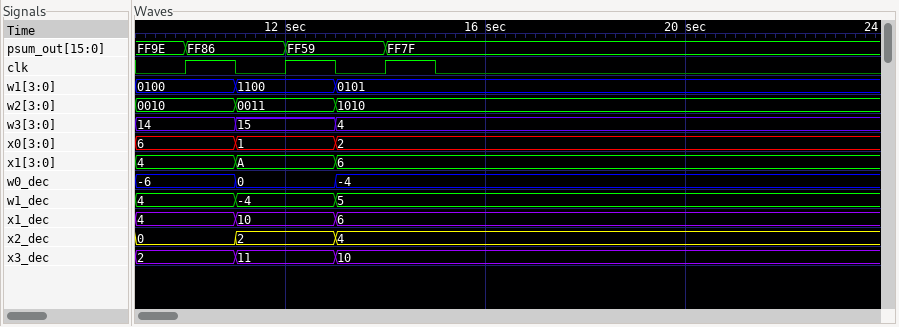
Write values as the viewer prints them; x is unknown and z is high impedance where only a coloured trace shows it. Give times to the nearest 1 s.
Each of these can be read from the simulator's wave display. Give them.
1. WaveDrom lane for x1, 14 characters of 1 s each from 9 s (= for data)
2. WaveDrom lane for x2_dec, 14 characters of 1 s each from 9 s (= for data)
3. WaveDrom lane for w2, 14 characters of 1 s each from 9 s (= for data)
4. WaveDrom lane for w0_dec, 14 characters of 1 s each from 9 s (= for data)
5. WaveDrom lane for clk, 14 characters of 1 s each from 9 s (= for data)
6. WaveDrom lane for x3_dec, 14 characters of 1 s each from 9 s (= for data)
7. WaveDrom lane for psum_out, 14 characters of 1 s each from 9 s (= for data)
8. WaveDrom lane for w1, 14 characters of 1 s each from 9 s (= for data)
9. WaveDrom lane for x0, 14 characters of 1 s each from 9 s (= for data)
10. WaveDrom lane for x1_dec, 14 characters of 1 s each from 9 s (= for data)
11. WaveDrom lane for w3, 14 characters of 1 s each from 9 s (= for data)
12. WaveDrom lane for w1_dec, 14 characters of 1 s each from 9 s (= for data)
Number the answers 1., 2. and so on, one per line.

1. {name: 'x1', wave: '=.=.=.........', data: '4 A 6'}
2. {name: 'x2_dec', wave: '=.=.=.........', data: '0 2 4'}
3. {name: 'w2', wave: '=.=.=.........', data: '0010 0011 1010'}
4. {name: 'w0_dec', wave: '=.=.=.........', data: '-6 0 -4'}
5. {name: 'clk', wave: '0101010.......'}
6. {name: 'x3_dec', wave: '=.=.=.........', data: '2 11 10'}
7. {name: 'psum_out', wave: '==.=.=........', data: 'FF9E FF86 FF59 FF7F'}
8. {name: 'w1', wave: '=.=.=.........', data: '0100 1100 0101'}
9. {name: 'x0', wave: '=.=.=.........', data: '6 1 2'}
10. {name: 'x1_dec', wave: '=.=.=.........', data: '4 10 6'}
11. {name: 'w3', wave: '=.=.=.........', data: '14 15 4'}
12. {name: 'w1_dec', wave: '=.=.=.........', data: '4 -4 5'}
